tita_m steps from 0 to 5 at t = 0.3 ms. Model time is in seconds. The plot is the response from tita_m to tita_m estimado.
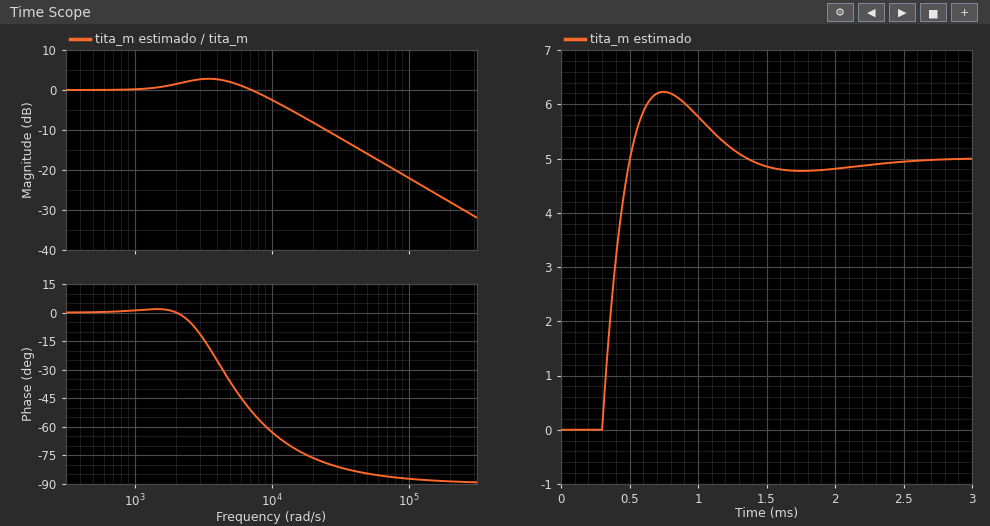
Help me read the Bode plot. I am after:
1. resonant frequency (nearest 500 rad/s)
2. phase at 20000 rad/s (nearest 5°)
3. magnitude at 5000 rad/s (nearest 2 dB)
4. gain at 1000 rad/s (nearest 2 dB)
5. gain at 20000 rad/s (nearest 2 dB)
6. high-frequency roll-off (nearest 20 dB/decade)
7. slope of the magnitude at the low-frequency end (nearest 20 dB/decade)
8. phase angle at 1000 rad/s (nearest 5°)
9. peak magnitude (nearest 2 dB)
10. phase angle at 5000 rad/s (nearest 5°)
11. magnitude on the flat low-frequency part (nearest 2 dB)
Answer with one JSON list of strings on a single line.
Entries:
["3500 rad/s", "-75°", "2 dB", "0 dB", "-8 dB", "-20 dB/decade", "0 dB/decade", "0°", "2 dB", "-35°", "0 dB"]
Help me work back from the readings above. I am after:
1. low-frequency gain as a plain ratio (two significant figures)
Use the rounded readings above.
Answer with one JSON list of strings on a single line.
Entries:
["1.0"]
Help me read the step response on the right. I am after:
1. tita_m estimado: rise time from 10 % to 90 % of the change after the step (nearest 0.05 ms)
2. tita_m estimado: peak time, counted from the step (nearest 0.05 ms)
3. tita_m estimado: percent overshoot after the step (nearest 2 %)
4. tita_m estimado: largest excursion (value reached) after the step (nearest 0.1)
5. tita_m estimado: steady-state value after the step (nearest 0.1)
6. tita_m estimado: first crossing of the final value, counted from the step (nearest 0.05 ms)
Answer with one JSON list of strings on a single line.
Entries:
["0.15 ms", "0.45 ms", "24 %", "6.2", "5.0", "0.20 ms"]
